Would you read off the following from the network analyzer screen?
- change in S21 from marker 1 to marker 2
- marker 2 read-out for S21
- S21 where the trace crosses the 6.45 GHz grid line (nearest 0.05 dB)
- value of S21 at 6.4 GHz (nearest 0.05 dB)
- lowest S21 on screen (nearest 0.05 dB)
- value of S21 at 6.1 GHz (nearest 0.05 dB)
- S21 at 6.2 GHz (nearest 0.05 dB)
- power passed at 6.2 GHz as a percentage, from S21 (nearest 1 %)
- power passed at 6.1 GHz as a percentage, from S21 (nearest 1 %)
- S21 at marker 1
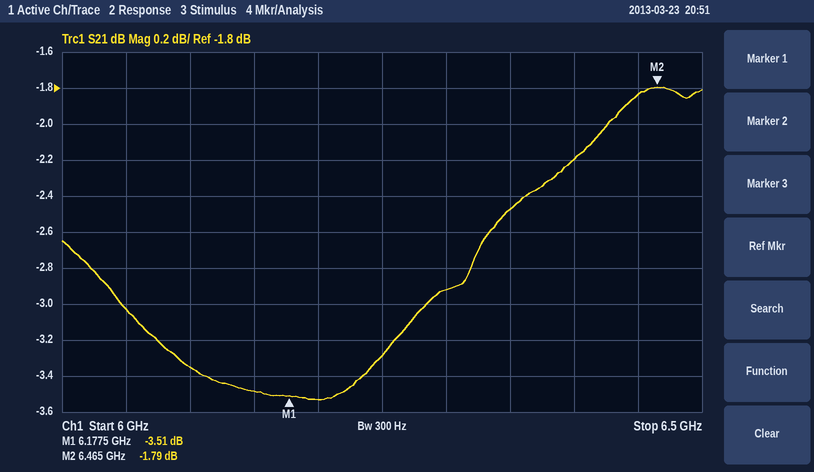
1.72 dB
-1.79 dB
-1.85 dB
-2.20 dB
-3.55 dB
-3.35 dB
-3.55 dB
44 %
46 %
-3.51 dB
